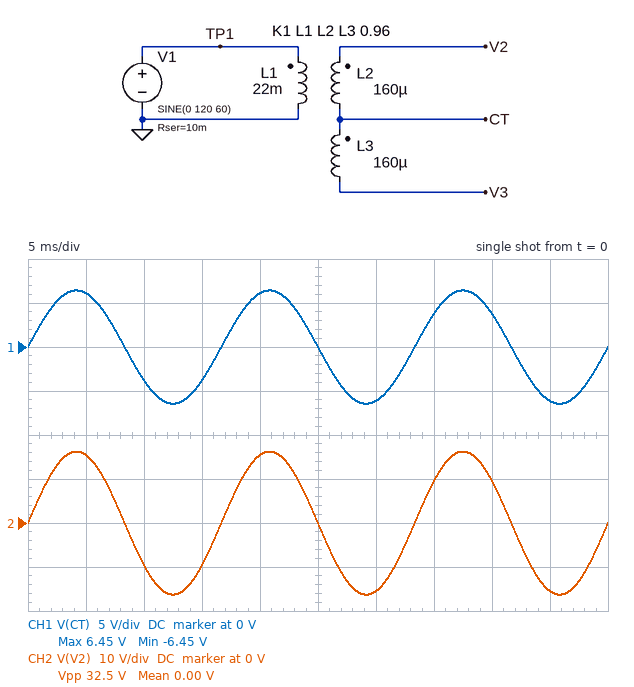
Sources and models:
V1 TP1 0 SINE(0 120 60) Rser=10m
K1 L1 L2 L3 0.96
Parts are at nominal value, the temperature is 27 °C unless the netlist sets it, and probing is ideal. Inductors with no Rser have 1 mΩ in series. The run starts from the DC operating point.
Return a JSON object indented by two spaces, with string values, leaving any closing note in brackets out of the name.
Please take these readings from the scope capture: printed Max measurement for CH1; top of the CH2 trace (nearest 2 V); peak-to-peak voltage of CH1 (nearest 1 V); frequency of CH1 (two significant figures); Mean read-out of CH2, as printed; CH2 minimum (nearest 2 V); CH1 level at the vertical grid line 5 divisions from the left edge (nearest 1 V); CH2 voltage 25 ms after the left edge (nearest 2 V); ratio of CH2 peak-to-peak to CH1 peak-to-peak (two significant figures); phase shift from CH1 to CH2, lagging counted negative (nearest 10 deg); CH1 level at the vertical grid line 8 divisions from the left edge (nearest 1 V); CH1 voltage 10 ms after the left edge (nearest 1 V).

{
  "printed Max measurement for CH1": "6.45 V",
  "top of the CH2 trace": "16 V",
  "peak-to-peak voltage of CH1": "13 V",
  "frequency of CH1": "60 Hz",
  "Mean read-out of CH2, as printed": "0.00 V",
  "CH2 minimum": "-16 V",
  "CH1 level at the vertical grid line 5 divisions from the left edge": "0 V",
  "CH2 voltage 25 ms after the left edge": "0 V",
  "ratio of CH2 peak-to-peak to CH1 peak-to-peak": "2.5",
  "phase shift from CH1 to CH2, lagging counted negative": "0 deg",
  "CH1 level at the vertical grid line 8 divisions from the left edge": "4 V",
  "CH1 voltage 10 ms after the left edge": "-4 V"
}
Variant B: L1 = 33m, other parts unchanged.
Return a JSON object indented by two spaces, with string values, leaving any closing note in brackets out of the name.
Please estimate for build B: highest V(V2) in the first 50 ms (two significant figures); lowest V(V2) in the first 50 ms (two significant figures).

{
  "highest V(V2) in the first 50 ms": "13 V",
  "lowest V(V2) in the first 50 ms": "-13 V"
}
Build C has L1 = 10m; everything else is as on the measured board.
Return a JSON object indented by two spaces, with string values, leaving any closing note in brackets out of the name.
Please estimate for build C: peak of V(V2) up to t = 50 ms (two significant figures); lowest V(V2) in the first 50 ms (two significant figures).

{
  "peak of V(V2) up to t = 50 ms": "24 V",
  "lowest V(V2) in the first 50 ms": "-24 V"
}
